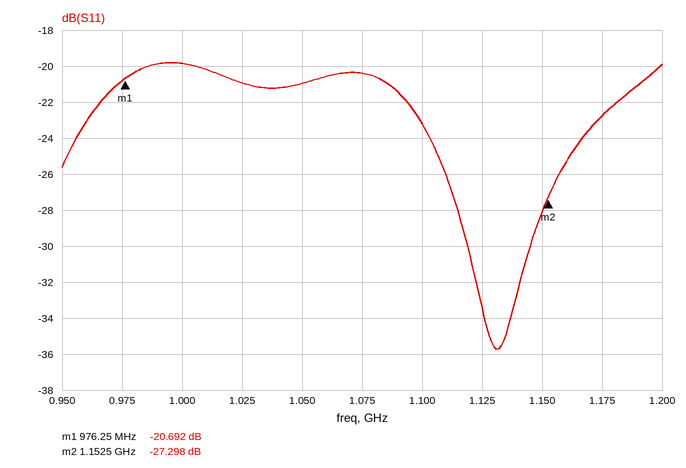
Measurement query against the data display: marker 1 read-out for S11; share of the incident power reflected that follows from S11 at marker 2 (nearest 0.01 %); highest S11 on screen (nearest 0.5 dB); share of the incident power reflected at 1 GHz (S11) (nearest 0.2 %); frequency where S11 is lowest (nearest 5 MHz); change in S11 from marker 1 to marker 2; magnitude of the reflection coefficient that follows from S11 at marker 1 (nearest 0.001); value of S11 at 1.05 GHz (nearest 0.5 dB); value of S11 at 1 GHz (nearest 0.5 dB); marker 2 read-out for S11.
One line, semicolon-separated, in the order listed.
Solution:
-20.692 dB; 0.19 %; -20.0 dB; 1.0 %; 1.130 GHz; -6.606 dB; 0.092; -21.0 dB; -20.0 dB; -27.298 dB
